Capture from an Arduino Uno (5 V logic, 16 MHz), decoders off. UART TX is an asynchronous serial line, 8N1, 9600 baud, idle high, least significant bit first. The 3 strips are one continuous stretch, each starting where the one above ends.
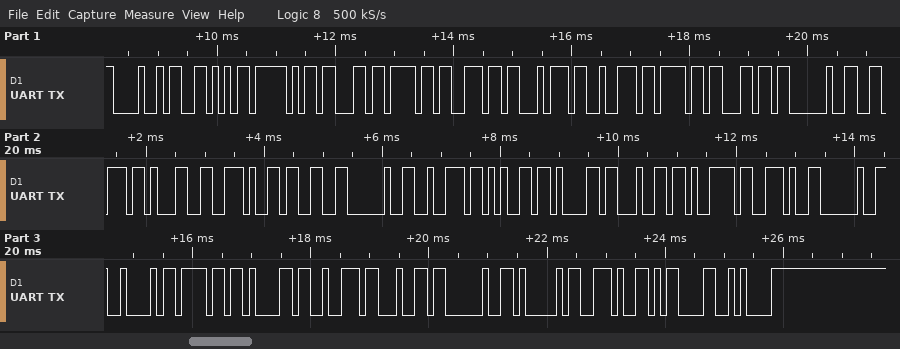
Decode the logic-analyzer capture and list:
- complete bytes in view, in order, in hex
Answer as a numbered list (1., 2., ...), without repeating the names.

1. 48 56 5F 63 6F 6E 74 72 6F 6C 20 76 31 2E 33 20 72 65 61 64 79 2E 20 42 6F 61 72 64 20 41 2E 0D 0A
